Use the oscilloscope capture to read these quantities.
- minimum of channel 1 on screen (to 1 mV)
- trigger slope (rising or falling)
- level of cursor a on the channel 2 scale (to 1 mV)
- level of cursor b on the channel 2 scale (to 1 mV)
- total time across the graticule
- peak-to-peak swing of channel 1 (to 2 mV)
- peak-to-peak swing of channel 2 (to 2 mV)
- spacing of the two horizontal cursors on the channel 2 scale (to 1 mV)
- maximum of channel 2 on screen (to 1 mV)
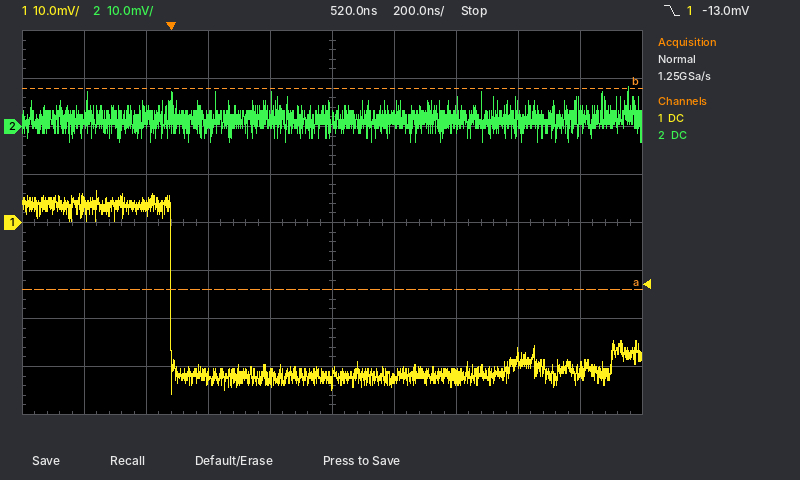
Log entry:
-36 mV
falling
-34 mV
8 mV
2 µs
42 mV
12 mV
42 mV
8 mV
